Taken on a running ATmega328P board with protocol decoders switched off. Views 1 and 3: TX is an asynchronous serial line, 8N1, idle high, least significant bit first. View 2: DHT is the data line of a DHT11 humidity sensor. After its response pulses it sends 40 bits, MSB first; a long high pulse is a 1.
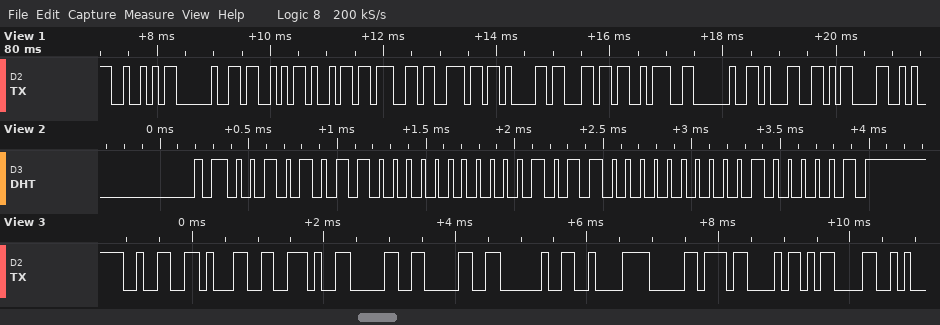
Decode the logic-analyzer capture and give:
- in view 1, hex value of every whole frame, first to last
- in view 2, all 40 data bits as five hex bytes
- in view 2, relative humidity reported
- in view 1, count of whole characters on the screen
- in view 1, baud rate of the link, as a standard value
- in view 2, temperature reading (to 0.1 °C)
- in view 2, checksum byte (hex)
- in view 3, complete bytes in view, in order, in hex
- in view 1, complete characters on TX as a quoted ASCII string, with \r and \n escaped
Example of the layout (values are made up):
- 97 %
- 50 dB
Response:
- 52 20 53 69 67 6E 61 6C 3A 20 31 0D
- 2B 00 16 00 41
- 43 %
- 12
- 9600 baud
- 22.0 °C
- 0x41
- 0x32 0x31 0x2E 0x30 0x30 0x20 0xC2 0xB0 0x43 0x0D
- "R Signal: 1\r"
